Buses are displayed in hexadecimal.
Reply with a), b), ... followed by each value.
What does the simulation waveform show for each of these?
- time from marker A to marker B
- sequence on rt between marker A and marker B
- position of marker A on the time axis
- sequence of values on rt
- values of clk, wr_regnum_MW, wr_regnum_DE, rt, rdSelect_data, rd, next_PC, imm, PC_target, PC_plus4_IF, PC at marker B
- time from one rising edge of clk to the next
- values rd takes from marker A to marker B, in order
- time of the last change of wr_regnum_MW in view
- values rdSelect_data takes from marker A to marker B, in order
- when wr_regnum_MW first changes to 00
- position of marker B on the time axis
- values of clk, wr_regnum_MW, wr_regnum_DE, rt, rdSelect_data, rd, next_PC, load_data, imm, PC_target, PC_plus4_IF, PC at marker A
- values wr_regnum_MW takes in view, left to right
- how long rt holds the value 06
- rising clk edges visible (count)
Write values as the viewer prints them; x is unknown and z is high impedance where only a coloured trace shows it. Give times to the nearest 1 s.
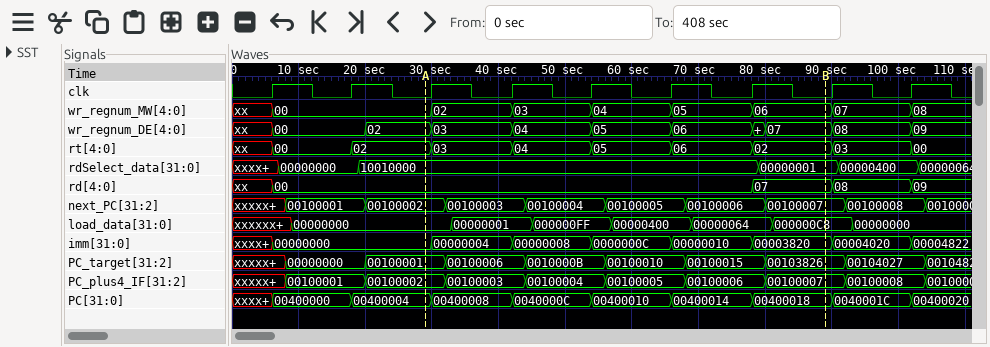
a) 60 s
b) 02, 03, 04, 05, 06, 02
c) 29 s
d) xx, 00, 02, 03, 04, 05, 06, 02, 03, 00
e) clk=0, wr_regnum_MW=06, wr_regnum_DE=07, rt=02, rdSelect_data=00000001, rd=07, next_PC=00100007, imm=00003820, PC_target=00103826, PC_plus4_IF=00100007, PC=00400018
f) 12 s
g) 00, 07
h) 102 s
i) 10010000, 00000001
j) 6 s
k) 89 s
l) clk=0, wr_regnum_MW=00, wr_regnum_DE=02, rt=02, rdSelect_data=10010000, rd=00, next_PC=00100002, load_data=00000000, imm=00000000, PC_target=00100001, PC_plus4_IF=00100002, PC=00400004
m) xx, 00, 02, 03, 04, 05, 06, 07, 08
n) 12 s
o) 9
